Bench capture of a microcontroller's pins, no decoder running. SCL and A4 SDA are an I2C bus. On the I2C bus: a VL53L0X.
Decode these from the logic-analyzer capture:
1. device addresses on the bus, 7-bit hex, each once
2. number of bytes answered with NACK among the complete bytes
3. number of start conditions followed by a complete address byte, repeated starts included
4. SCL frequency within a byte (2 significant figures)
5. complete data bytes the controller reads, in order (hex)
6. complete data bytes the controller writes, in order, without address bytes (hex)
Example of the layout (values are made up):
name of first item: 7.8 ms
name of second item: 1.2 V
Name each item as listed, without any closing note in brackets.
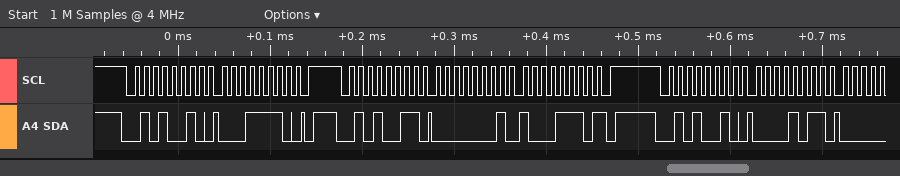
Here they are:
device addresses on the bus, 7-bit hex, each once: 0x29
number of bytes answered with NACK among the complete bytes: 1
number of start conditions followed by a complete address byte, repeated starts included: 3
SCL frequency within a byte: 100 kHz
complete data bytes the controller reads, in order: 01 8E
complete data bytes the controller writes, in order, without address bytes: 1E 0B
